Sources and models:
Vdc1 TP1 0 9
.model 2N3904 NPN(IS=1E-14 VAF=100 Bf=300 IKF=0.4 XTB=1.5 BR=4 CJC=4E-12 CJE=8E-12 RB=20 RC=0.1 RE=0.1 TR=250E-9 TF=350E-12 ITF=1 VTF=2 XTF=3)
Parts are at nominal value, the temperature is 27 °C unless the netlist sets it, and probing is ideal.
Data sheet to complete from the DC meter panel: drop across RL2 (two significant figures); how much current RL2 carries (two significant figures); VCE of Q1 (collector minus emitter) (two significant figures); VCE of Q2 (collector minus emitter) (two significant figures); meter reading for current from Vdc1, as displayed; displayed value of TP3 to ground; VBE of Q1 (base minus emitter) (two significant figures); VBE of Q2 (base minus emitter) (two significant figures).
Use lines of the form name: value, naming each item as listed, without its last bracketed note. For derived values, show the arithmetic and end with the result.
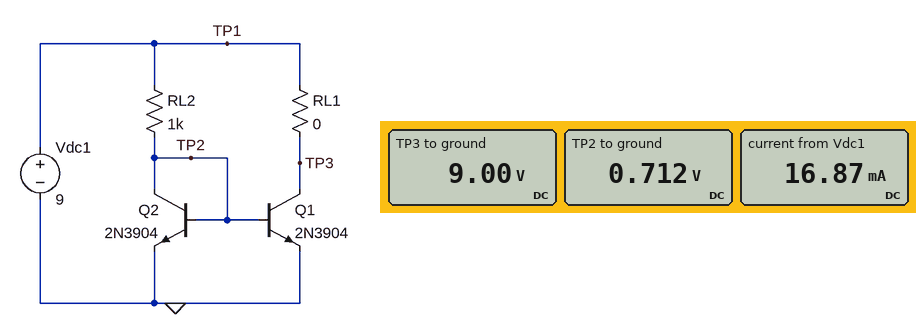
drop across RL2: 9 V - 712 mV = 8.3 V
how much current RL2 carries: (9 V - 712 mV) / 1 kΩ = 8.3 mA
VCE of Q1 (collector minus emitter): 9 V = 9.0 V
VCE of Q2 (collector minus emitter): 712 mV = 710 mV
meter reading for current from Vdc1, as displayed: 16.87 mA
displayed value of TP3 to ground: 9.00 V
VBE of Q1 (base minus emitter): 712 mV = 710 mV
VBE of Q2 (base minus emitter): 712 mV = 710 mV
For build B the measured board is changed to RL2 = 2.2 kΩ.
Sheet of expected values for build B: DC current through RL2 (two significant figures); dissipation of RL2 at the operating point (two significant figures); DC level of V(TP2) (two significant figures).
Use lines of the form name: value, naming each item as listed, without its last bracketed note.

DC current through RL2: 3.8 mA
dissipation of RL2 at the operating point: 31 mW
DC level of V(TP2): 690 mV
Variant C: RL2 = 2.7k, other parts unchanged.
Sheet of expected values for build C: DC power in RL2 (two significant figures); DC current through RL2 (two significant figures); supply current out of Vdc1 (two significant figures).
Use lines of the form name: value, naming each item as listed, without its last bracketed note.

DC power in RL2: 26 mW
DC current through RL2: 3.1 mA
supply current out of Vdc1: 7.6 mA
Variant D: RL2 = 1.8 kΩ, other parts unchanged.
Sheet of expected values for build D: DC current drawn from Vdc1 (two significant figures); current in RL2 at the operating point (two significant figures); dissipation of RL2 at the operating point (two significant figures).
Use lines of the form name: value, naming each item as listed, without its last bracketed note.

DC current drawn from Vdc1: 11 mA
current in RL2 at the operating point: 4.6 mA
dissipation of RL2 at the operating point: 38 mW
